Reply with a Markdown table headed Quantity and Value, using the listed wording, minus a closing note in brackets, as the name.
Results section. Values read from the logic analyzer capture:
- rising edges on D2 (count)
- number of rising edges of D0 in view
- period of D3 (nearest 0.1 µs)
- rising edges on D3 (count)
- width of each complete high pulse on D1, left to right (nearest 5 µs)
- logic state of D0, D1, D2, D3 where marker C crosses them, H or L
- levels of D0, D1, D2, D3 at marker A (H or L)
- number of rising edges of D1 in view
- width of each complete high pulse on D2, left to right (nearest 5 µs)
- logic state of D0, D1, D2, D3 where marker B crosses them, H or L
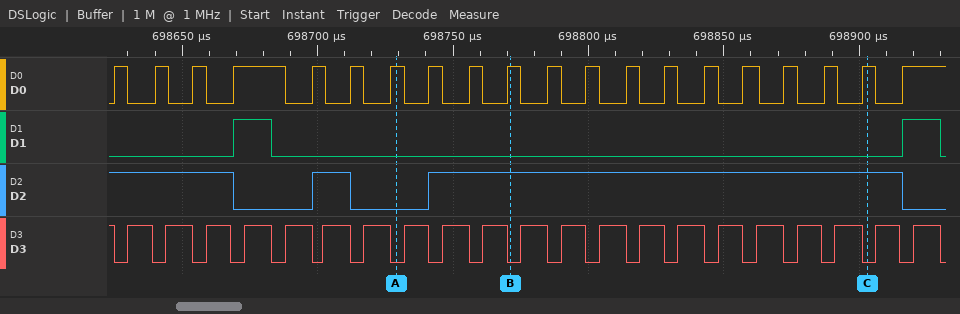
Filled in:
| Quantity | Value |
|---|---|
| rising edges on D2 | 2 |
| number of rising edges of D0 in view | 20 |
| period of D3 | 14.5 µs |
| rising edges on D3 | 21 |
| width of each complete high pulse on D1, left to right | 15 µs, 15 µs |
| logic state of D0, D1, D2, D3 where marker C crosses them, H or L | D0=H, D1=L, D2=H, D3=L |
| levels of D0, D1, D2, D3 at marker A | D0=H, D1=L, D2=L, D3=L |
| number of rising edges of D1 in view | 2 |
| width of each complete high pulse on D2, left to right | 15 µs, 175 µs |
| logic state of D0, D1, D2, D3 where marker B crosses them, H or L | D0=H, D1=L, D2=H, D3=L |
